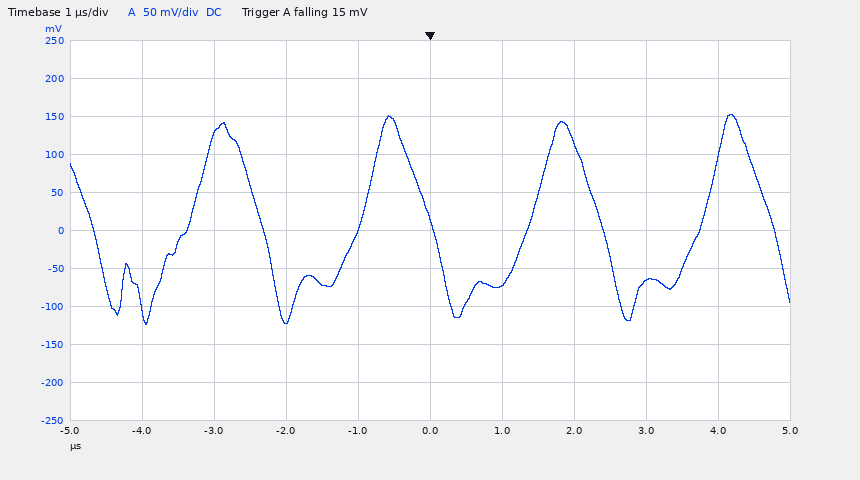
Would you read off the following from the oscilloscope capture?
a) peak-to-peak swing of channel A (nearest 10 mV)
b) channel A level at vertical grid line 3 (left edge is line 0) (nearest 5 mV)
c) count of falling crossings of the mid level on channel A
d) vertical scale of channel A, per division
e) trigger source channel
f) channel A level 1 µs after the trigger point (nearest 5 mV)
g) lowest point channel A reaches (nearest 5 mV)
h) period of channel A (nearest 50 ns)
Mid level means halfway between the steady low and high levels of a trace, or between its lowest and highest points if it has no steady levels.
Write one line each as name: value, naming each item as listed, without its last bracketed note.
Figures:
peak-to-peak swing of channel A: 280 mV
channel A level at vertical grid line 3 (left edge is line 0): -120 mV
count of falling crossings of the mid level on channel A: 5
vertical scale of channel A, per division: 50 mV
trigger source channel: channel A
channel A level 1 µs after the trigger point: -70 mV
lowest point channel A reaches: -125 mV
period of channel A: 2.35 µs
